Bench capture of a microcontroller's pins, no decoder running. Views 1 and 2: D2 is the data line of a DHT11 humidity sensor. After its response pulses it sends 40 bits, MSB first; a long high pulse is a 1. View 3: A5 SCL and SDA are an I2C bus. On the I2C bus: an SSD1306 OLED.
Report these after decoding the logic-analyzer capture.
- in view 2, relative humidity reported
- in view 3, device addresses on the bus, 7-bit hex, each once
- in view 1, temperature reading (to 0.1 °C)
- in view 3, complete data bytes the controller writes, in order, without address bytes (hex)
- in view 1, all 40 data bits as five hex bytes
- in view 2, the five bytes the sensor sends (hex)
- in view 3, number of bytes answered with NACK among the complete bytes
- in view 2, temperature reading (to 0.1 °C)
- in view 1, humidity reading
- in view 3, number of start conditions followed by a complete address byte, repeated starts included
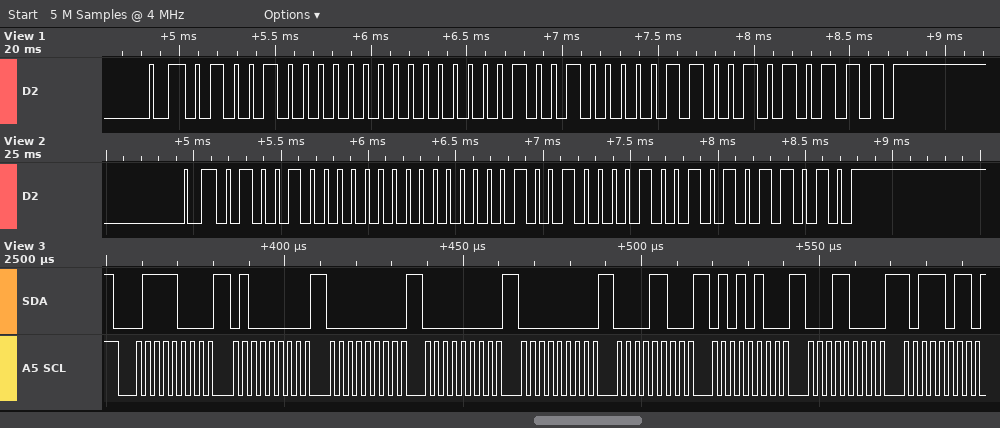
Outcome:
72 %
0x3C
9.6 °C
40 00 00 00 0C 54 18 BB
48 00 09 06 57
48 00 09 09 5A
0
9.9 °C
72 %
1
